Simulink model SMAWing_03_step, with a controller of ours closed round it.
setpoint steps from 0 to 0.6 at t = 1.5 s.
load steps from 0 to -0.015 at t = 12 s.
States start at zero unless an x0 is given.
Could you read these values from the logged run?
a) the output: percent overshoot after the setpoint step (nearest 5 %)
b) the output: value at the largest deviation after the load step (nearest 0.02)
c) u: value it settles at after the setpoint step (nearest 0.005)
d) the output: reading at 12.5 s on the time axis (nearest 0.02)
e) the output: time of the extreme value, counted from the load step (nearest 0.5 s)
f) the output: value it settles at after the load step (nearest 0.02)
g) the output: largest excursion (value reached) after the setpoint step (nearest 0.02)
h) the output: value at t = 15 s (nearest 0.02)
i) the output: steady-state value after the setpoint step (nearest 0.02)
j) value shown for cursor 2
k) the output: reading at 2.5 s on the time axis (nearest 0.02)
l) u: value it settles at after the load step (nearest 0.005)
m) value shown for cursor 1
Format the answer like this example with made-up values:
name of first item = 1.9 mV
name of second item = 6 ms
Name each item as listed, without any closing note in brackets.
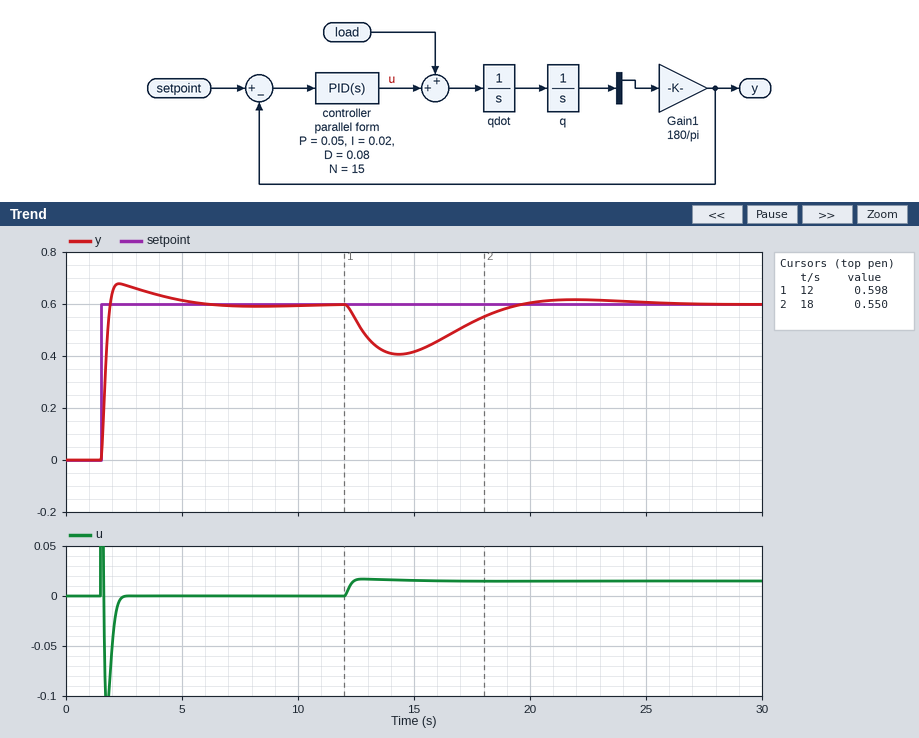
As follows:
the output: percent overshoot after the setpoint step = 15 %
the output: value at the largest deviation after the load step = 0.40
u: value it settles at after the setpoint step = 0.000
the output: reading at 12.5 s on the time axis = 0.54
the output: time of the extreme value, counted from the load step = 2.5 s
the output: value it settles at after the load step = 0.60
the output: largest excursion (value reached) after the setpoint step = 0.68
the output: value at t = 15 s = 0.42
the output: steady-state value after the setpoint step = 0.60
value shown for cursor 2 = 0.550
the output: reading at 2.5 s on the time axis = 0.68
u: value it settles at after the load step = 0.015
value shown for cursor 1 = 0.598
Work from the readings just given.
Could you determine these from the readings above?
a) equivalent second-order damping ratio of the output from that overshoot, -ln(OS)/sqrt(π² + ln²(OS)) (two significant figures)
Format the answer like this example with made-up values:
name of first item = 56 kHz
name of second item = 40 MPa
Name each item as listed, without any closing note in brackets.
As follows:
equivalent second-order damping ratio of the output from that overshoot, -ln(OS)/sqrt(π² + ln²(OS)) = 0.52
